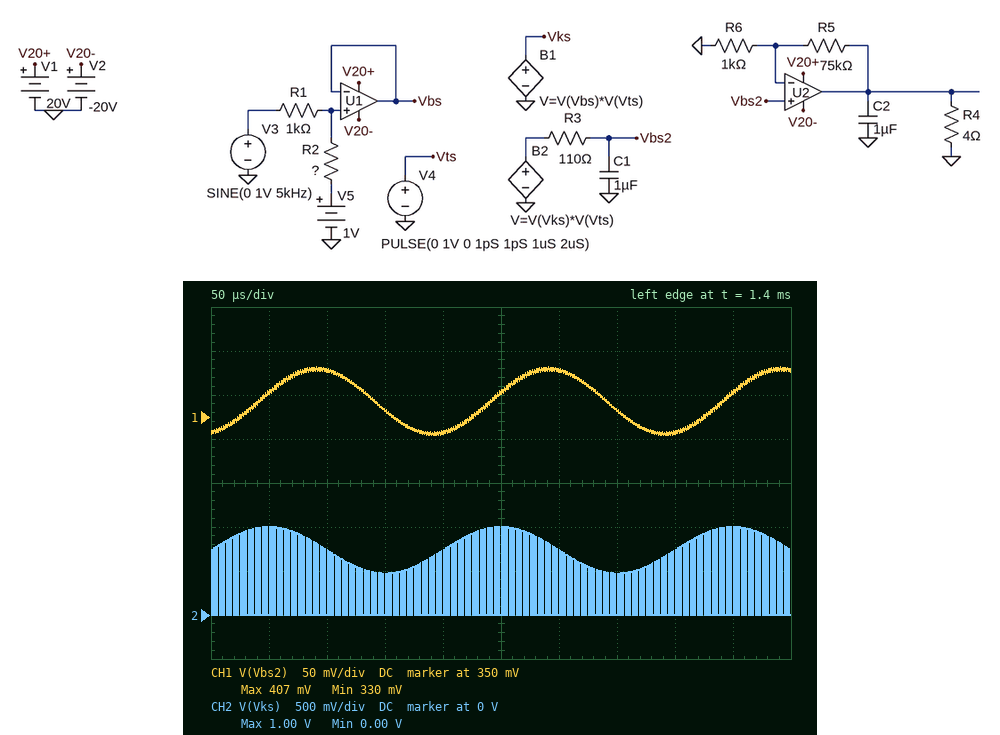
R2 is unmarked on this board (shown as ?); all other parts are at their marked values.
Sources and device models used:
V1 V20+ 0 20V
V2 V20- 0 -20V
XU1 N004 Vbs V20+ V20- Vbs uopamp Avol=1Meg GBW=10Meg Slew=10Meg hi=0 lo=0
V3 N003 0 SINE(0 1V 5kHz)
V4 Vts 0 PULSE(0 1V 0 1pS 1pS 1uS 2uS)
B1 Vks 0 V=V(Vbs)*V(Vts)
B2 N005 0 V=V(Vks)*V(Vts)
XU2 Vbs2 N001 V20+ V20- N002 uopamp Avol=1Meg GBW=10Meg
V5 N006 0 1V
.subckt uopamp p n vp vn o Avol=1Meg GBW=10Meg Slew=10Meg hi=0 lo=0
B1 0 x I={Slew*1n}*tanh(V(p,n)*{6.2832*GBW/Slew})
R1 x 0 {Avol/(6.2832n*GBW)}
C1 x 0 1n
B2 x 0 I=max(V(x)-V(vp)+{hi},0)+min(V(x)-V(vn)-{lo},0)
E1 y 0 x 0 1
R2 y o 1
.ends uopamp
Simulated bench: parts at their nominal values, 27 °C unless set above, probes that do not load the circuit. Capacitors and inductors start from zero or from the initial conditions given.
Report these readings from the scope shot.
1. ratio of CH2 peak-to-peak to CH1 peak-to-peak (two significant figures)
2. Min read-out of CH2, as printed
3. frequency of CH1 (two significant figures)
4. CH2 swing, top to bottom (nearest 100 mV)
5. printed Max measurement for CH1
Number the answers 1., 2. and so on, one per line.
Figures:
1. 13
2. 0.00 V
3. 5.0 kHz
4. 1.0 V
5. 407 mV
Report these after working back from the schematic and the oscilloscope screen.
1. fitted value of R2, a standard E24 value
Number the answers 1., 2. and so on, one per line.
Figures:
1. 360 Ω
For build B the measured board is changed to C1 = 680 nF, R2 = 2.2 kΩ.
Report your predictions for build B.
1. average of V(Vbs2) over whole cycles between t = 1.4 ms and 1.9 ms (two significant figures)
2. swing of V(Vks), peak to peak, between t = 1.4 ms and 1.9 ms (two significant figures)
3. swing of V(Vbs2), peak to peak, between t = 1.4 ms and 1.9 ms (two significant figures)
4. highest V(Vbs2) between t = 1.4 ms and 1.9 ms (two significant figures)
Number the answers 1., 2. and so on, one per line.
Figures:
1. 160 mV
2. 1.4 V
3. 270 mV
4. 290 mV
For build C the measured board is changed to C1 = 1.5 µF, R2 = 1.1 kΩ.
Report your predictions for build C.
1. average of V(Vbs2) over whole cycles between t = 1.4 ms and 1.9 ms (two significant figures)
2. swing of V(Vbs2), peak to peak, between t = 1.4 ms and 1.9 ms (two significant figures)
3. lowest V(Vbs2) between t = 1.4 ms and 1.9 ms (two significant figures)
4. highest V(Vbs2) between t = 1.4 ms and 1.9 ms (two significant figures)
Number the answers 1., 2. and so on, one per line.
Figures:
1. 240 mV
2. 100 mV
3. 190 mV
4. 290 mV
